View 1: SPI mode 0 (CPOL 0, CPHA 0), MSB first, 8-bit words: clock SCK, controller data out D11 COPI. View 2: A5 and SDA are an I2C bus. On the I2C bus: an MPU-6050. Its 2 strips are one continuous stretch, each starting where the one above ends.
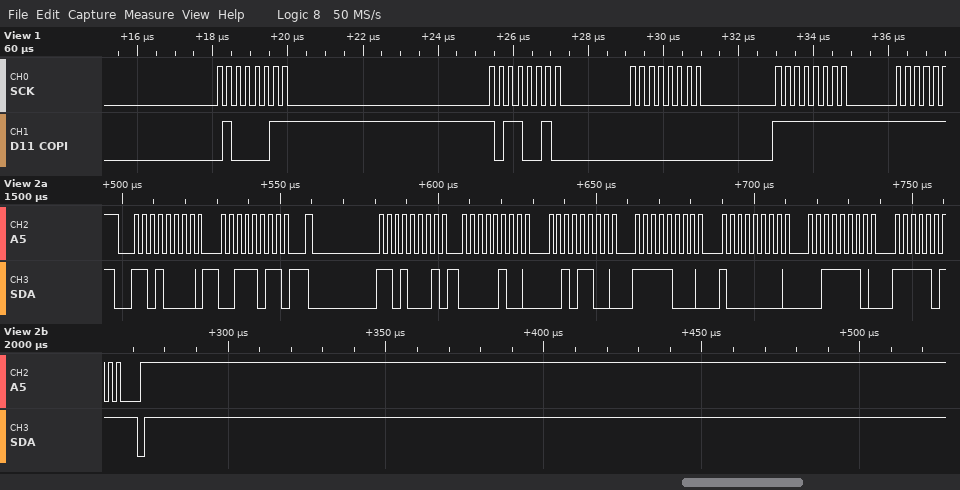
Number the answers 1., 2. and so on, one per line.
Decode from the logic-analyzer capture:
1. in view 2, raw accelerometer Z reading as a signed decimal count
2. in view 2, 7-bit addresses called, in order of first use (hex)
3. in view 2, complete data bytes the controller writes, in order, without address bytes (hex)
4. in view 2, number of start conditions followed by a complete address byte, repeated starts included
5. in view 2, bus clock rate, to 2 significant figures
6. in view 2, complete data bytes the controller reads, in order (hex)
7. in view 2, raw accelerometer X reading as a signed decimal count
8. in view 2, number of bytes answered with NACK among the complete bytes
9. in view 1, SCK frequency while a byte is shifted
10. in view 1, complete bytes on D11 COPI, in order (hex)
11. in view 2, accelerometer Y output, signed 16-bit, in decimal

1. 16123
2. 0x68
3. 3B
4. 2
5. 400 kHz
6. 04 2C F8 80 3E FB
7. 1068
8. 1
9. 4 MHz
10. 43 B2 00 FF
11. -1920
